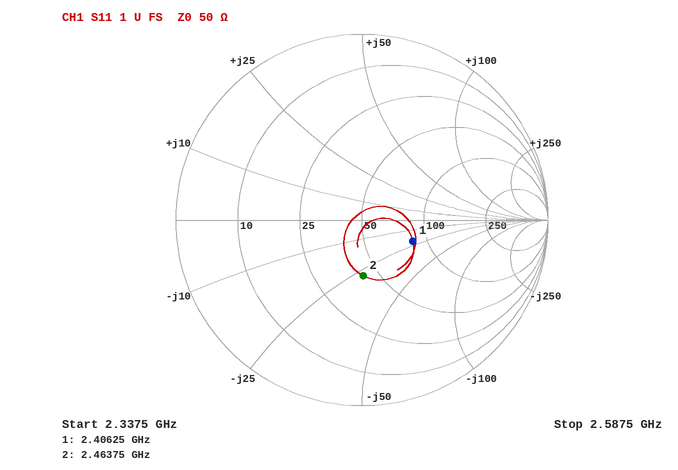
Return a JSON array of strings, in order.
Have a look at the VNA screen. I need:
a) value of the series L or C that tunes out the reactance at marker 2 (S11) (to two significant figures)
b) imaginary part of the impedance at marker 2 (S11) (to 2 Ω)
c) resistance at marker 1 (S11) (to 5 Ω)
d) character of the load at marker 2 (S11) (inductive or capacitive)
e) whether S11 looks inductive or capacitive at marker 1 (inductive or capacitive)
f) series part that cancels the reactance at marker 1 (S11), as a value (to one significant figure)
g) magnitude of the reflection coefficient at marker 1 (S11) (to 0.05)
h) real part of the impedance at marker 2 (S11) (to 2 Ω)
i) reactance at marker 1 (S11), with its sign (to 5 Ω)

["1.8 nH", "-28 Ω", "85 Ω", "capacitive", "capacitive", "1 nH", "0.30", "42 Ω", "-20 Ω"]
